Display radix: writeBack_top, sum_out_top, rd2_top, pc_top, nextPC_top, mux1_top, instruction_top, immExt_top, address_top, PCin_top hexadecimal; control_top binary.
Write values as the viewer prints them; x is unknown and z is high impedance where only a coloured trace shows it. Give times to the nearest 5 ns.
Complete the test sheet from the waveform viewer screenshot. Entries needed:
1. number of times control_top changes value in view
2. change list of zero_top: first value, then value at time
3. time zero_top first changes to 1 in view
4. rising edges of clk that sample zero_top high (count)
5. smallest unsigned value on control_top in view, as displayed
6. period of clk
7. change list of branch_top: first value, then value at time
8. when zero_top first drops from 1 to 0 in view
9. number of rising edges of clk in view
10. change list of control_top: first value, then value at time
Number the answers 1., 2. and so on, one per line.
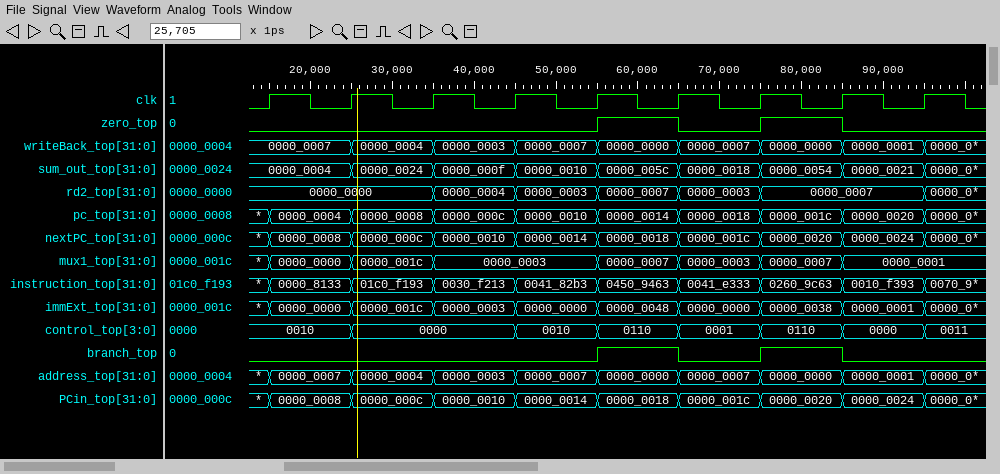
1. 7
2. 0, 1 at 55 ns, 0 at 65 ns, 1 at 75 ns, 0 at 85 ns
3. 55 ns
4. 2
5. 0000
6. 10 ns
7. 0, 1 at 55 ns, 0 at 65 ns, 1 at 75 ns, 0 at 85 ns
8. 65 ns
9. 9
10. 0010, 0000 at 25 ns, 0010 at 45 ns, 0110 at 55 ns, 0001 at 65 ns, 0110 at 75 ns, 0000 at 85 ns, 0011 at 95 ns
